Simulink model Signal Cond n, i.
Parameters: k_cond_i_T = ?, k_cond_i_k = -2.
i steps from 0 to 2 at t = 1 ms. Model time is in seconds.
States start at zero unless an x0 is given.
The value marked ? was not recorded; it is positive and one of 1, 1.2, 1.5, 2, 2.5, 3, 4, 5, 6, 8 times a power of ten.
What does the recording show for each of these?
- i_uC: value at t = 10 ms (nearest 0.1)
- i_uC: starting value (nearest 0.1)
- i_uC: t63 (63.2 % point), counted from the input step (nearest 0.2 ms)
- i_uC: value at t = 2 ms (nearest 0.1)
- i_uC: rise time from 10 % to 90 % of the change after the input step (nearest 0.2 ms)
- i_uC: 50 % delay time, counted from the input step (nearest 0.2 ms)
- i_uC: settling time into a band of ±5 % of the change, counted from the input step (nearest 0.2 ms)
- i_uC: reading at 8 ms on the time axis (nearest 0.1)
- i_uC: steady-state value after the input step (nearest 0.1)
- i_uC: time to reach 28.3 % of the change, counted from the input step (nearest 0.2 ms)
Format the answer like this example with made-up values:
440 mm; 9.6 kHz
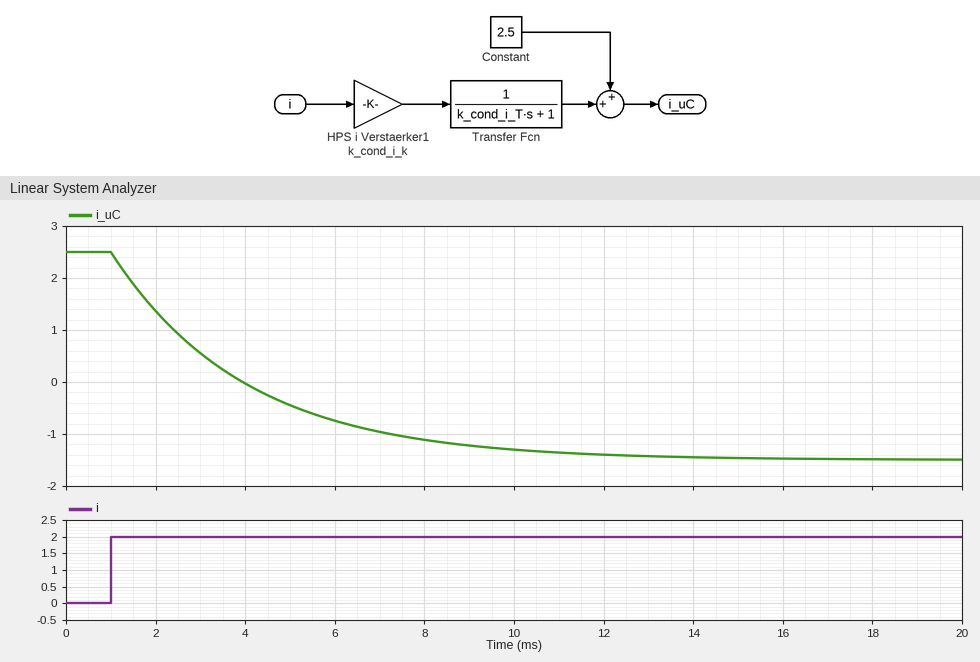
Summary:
-1.3; 2.5; 3.0 ms; 1.4; 6.6 ms; 2.0 ms; 9.0 ms; -1.1; -1.5; 1.0 ms
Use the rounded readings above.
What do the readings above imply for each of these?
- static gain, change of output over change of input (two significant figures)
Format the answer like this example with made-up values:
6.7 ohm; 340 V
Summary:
-2.0
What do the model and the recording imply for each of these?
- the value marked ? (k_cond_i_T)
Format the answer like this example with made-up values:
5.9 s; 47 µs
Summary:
0.003
